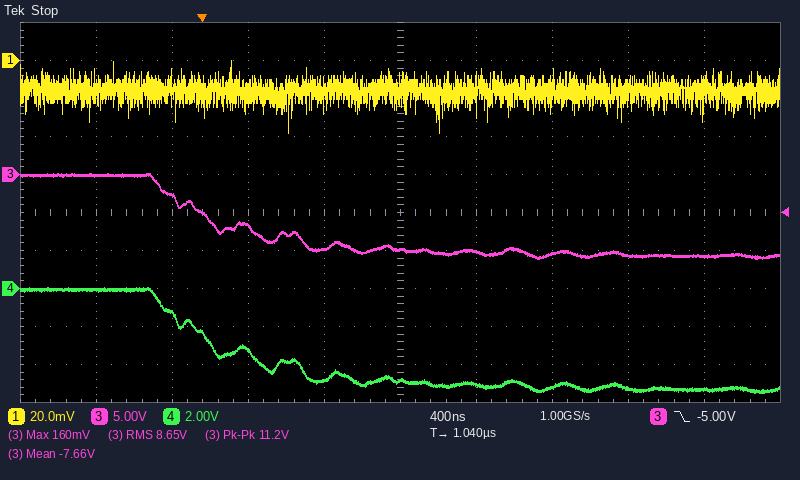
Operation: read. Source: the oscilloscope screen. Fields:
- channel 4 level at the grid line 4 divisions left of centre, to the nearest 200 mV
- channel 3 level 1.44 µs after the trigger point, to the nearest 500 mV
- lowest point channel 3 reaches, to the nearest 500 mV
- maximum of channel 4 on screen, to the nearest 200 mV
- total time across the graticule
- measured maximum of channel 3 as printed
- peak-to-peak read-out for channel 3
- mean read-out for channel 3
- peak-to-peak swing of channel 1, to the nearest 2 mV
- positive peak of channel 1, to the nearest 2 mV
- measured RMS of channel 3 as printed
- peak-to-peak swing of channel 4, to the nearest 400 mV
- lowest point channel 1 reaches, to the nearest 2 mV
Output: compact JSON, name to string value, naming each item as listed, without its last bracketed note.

{"channel 4 level at the grid line 4 divisions left of centre, to the nearest 200 mV": "0.0 V", "channel 3 level 1.44 µs after the trigger point, to the nearest 500 mV": "-10.0 V", "lowest point channel 3 reaches, to the nearest 500 mV": "-11.0 V", "maximum of channel 4 on screen, to the nearest 200 mV": "0.0 V", "total time across the graticule": "4 µs", "measured maximum of channel 3 as printed": "160 mV", "peak-to-peak read-out for channel 3": "11.2 V", "mean read-out for channel 3": "-7.66 V", "peak-to-peak swing of channel 1, to the nearest 2 mV": "38 mV", "positive peak of channel 1, to the nearest 2 mV": "0 mV", "measured RMS of channel 3 as printed": "8.65 V", "peak-to-peak swing of channel 4, to the nearest 400 mV": "5.6 V", "lowest point channel 1 reaches, to the nearest 2 mV": "-38 mV"}
